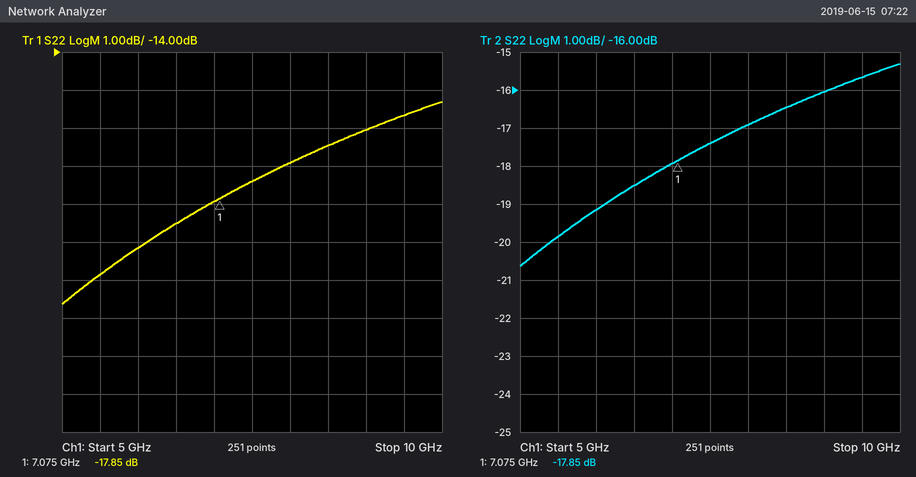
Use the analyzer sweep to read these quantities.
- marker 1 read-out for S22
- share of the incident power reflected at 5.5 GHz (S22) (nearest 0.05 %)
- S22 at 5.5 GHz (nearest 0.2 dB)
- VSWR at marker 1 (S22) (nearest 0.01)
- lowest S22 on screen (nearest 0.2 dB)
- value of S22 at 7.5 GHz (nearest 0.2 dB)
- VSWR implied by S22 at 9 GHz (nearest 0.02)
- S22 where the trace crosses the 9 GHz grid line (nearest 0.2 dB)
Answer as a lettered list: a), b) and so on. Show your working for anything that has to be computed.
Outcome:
a) -17.85 dB
b) 10^(-19.8/10) ≈ 1.05 %
c) -19.8 dB
d) (1 + 0.1281)/(1 − 0.1281) ≈ 1.29
e) -20.6 dB
f) -17.4 dB
g) |Γ| = 10^(-16/20) = 0.1585; VSWR = (1 + 0.1585)/(1 − 0.1585) ≈ 1.38
h) -16.0 dB
